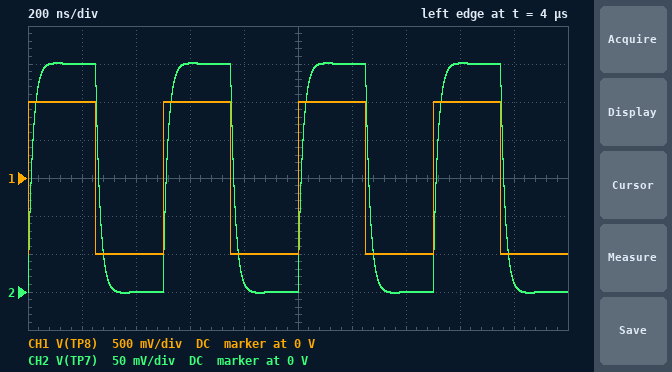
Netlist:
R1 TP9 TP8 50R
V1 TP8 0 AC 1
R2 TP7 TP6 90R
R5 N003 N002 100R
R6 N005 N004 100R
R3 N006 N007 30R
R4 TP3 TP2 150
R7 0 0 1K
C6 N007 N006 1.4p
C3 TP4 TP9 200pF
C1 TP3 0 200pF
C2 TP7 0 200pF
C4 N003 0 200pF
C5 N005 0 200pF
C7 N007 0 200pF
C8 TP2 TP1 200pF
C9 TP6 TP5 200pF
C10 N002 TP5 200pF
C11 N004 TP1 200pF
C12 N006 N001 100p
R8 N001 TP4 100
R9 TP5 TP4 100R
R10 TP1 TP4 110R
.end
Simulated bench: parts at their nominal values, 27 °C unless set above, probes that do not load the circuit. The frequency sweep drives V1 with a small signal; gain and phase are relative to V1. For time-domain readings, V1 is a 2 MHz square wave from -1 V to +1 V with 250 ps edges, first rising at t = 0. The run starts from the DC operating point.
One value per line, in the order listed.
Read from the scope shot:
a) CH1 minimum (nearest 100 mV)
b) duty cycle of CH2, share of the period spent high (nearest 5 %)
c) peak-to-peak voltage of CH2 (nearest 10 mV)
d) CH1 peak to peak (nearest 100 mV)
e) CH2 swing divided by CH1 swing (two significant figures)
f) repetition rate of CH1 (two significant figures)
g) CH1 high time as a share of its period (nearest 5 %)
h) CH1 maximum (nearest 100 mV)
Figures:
-1.0 V
50 %
300 mV
2.0 V
0.15
2.0 MHz
50 %
1.0 V
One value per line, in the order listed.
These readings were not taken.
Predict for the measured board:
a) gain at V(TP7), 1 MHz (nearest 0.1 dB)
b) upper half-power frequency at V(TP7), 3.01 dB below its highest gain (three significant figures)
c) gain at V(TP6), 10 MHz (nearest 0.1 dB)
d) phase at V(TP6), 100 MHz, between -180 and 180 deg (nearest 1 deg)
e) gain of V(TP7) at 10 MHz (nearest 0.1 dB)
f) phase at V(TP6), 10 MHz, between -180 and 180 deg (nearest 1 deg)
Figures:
-16.5 dB
9.68 MHz
-16.1 dB
0 deg
-19.6 dB
1 deg
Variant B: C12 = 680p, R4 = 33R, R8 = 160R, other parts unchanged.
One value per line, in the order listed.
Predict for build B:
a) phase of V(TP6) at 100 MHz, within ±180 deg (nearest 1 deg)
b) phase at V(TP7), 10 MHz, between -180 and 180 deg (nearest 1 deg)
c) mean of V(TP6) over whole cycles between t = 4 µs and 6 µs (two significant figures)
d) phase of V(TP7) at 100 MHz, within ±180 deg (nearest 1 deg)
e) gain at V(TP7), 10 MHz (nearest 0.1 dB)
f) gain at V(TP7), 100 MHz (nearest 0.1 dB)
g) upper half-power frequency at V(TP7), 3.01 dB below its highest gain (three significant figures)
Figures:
1 deg
-43 deg
130 mV
-84 deg
-20.3 dB
-36.9 dB
10.7 MHz
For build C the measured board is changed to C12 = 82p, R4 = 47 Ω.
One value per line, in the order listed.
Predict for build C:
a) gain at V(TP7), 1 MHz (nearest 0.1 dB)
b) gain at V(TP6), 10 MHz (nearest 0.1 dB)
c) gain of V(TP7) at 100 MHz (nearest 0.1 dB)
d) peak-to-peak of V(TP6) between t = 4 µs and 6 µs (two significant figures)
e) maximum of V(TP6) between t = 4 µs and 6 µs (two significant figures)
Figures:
-16.4 dB
-16.2 dB
-37.3 dB
320 mV
310 mV
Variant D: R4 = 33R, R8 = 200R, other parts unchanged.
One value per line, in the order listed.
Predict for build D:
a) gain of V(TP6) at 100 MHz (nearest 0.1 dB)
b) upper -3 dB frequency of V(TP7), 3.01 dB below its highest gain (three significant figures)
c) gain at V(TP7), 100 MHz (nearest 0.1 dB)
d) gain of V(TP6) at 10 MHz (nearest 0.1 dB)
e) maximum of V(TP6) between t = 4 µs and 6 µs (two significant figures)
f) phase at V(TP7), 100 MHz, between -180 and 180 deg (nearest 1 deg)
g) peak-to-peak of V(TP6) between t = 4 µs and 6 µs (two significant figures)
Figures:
-15.6 dB
9.32 MHz
-36.7 dB
-16.2 dB
330 mV
-84 deg
370 mV
